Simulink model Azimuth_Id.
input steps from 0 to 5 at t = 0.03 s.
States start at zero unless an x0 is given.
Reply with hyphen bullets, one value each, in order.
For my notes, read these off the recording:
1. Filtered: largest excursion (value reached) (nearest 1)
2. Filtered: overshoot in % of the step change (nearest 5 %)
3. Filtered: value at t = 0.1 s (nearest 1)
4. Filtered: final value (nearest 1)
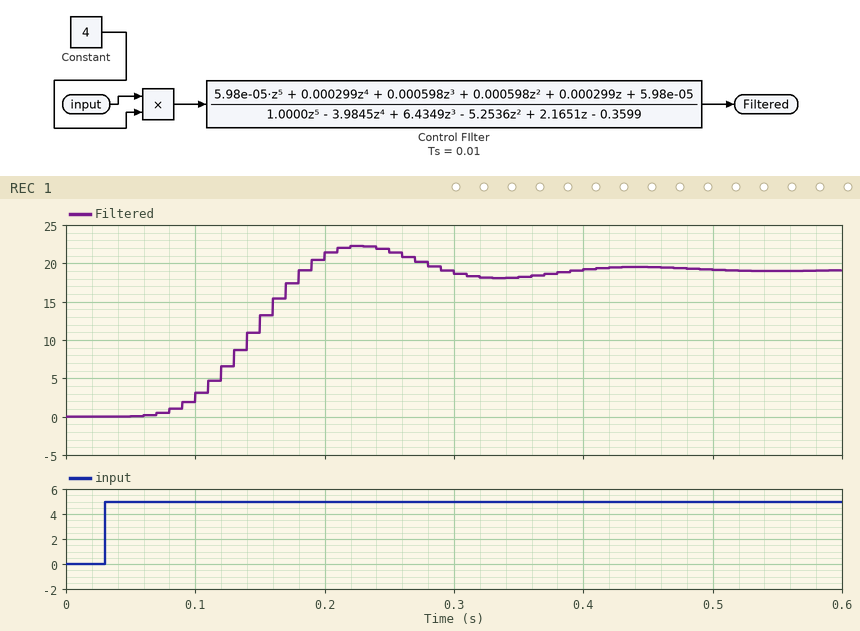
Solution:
- 22
- 15 %
- 3
- 19
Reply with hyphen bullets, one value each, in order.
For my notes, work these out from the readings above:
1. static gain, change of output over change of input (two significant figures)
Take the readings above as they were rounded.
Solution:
- 3.8
